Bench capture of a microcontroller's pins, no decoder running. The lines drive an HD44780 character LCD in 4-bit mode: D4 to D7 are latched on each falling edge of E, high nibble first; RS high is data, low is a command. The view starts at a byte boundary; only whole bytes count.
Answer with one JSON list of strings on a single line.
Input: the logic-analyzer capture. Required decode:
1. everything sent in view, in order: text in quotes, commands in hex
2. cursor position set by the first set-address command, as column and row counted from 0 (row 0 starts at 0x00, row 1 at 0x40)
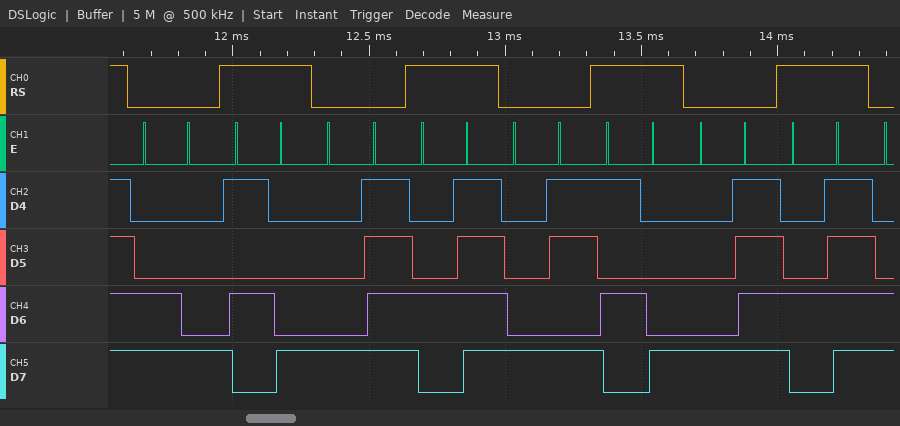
["0xC8 \"X\" 0x8F \"O\" 0x8B \"X\" 0x8F \"O\"", "column 8, row 1"]
